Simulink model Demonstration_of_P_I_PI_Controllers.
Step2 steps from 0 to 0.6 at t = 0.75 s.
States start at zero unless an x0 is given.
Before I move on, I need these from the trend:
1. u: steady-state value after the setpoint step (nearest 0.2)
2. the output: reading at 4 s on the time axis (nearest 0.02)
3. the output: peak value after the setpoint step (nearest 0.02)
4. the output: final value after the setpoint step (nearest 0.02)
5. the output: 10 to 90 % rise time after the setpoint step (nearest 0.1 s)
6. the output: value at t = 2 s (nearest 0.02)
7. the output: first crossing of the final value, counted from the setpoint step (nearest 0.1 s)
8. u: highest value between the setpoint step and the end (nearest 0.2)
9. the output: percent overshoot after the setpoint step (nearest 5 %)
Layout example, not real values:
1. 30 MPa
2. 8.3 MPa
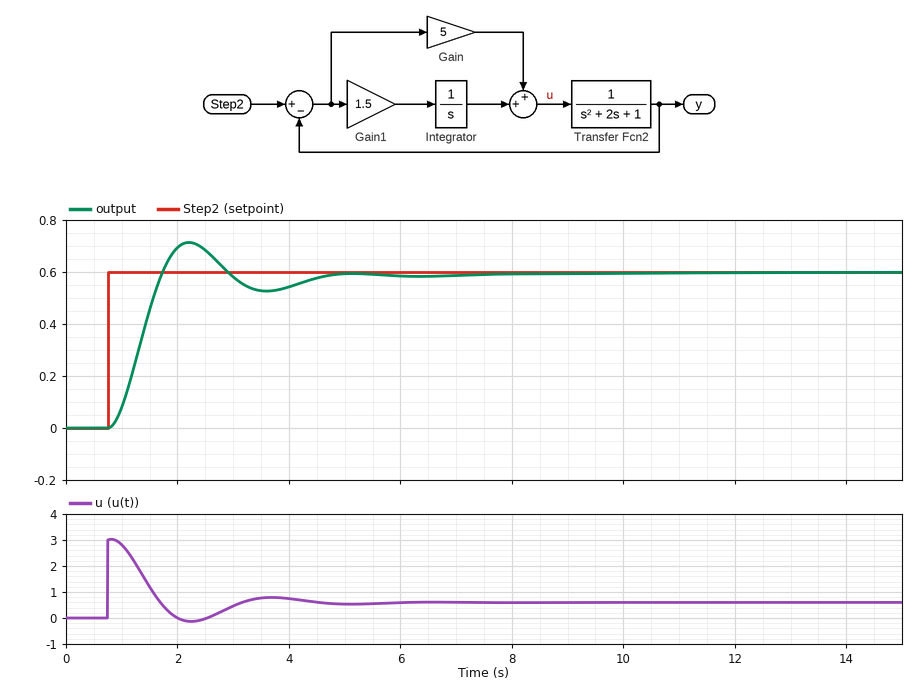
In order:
1. 0.6
2. 0.54
3. 0.72
4. 0.60
5. 0.7 s
6. 0.70
7. 1.0 s
8. 3.0
9. 20 %
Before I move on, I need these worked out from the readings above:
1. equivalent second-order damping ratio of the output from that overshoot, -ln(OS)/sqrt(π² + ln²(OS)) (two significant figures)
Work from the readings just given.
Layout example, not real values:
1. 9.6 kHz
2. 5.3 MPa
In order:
1. 0.46
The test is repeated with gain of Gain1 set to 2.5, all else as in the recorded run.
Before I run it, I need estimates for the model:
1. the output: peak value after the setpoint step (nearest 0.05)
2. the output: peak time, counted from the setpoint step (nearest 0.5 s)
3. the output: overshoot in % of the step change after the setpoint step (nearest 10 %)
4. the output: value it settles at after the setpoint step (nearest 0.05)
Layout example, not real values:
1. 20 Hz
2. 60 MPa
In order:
1. 0.75
2. 1.5 s
3. 30 %
4. 0.60
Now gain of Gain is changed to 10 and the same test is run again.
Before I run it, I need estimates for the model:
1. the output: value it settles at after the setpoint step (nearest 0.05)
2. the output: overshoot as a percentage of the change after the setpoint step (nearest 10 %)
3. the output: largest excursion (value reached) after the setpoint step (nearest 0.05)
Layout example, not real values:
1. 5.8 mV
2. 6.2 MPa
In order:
1. 0.60
2. 30 %
3. 0.80
